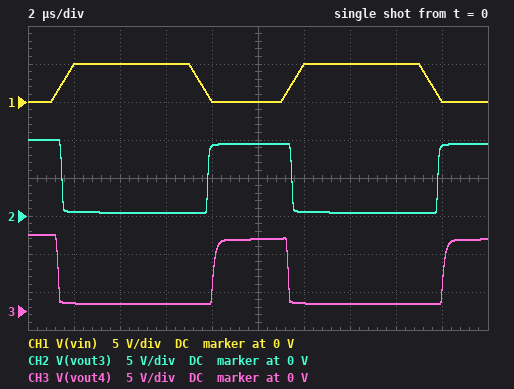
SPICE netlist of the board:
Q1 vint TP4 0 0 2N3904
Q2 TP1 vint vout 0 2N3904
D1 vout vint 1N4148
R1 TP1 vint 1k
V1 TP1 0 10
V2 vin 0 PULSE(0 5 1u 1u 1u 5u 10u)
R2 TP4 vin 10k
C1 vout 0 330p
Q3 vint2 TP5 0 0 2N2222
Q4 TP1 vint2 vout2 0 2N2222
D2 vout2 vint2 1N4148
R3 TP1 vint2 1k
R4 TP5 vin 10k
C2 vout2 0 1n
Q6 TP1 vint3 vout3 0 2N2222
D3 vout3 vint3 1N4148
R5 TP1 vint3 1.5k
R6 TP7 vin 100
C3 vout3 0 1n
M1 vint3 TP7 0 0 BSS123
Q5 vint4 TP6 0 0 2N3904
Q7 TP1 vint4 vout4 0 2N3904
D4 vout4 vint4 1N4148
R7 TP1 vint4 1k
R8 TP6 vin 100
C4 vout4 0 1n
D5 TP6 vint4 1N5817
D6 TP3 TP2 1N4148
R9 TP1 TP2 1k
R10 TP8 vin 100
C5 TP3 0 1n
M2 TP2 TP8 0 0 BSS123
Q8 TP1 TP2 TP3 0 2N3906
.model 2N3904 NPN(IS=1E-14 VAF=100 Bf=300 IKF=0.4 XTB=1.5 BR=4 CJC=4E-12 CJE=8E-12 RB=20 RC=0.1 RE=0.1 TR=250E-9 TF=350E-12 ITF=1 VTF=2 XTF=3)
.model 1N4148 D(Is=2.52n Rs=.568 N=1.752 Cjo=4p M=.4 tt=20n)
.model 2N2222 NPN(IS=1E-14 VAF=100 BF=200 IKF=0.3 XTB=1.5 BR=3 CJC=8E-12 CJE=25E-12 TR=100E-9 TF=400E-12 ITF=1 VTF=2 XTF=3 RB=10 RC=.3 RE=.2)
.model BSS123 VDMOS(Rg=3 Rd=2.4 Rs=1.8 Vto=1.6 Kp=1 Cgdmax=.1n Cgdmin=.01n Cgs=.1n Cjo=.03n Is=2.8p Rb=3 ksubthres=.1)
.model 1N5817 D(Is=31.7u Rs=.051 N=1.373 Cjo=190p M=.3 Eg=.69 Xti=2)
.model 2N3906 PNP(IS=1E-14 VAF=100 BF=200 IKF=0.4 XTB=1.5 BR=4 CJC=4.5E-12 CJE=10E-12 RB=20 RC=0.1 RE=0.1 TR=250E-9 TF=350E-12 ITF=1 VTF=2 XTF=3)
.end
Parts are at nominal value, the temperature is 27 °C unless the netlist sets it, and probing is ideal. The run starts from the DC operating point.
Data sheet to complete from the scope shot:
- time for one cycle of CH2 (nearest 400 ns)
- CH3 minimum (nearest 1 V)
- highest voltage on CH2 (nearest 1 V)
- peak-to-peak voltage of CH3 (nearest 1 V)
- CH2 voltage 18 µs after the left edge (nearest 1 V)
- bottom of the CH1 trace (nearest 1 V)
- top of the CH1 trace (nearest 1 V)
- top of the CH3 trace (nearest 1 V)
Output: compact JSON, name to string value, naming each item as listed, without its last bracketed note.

{"time for one cycle of CH2": "10.0 µs", "CH3 minimum": "1 V", "highest voltage on CH2": "10 V", "peak-to-peak voltage of CH3": "9 V", "CH2 voltage 18 µs after the left edge": "9 V", "bottom of the CH1 trace": "0 V", "top of the CH1 trace": "5 V", "top of the CH3 trace": "10 V"}
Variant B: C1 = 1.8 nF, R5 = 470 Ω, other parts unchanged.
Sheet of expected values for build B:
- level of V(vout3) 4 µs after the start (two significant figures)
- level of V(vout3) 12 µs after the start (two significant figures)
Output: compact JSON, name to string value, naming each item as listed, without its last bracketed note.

{"level of V(vout3) 4 µs after the start": "500 mV", "level of V(vout3) 12 µs after the start": "600 mV"}
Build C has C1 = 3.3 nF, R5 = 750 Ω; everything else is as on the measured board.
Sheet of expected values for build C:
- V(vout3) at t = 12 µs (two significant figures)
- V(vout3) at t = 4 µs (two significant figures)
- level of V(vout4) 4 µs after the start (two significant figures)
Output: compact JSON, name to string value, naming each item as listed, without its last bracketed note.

{"V(vout3) at t = 12 µs": "560 mV", "V(vout3) at t = 4 µs": "470 mV", "level of V(vout4) 4 µs after the start": "920 mV"}
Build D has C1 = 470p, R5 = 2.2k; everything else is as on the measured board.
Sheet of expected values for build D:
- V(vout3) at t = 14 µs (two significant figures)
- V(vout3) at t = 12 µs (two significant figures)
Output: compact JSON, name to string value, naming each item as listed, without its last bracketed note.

{"V(vout3) at t = 14 µs": "430 mV", "V(vout3) at t = 12 µs": "520 mV"}
